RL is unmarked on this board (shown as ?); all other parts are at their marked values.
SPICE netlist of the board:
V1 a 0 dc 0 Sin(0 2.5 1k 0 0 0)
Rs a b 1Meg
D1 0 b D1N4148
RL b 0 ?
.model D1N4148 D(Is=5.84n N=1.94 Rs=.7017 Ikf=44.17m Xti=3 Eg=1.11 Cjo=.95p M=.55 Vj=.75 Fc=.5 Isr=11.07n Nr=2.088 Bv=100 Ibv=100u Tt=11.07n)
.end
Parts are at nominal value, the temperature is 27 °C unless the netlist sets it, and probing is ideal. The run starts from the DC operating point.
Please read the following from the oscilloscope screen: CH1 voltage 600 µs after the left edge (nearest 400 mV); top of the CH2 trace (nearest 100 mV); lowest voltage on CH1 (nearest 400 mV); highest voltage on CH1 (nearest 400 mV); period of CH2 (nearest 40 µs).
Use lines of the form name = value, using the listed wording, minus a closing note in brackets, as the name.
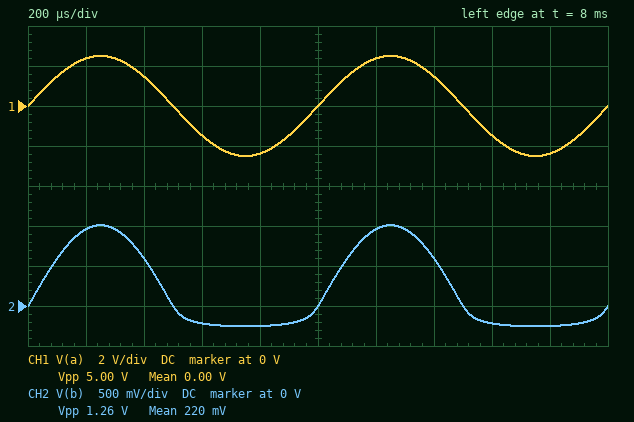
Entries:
CH1 voltage 600 µs after the left edge = -1.6 V
top of the CH2 trace = 1.0 V
lowest voltage on CH1 = -2.4 V
highest voltage on CH1 = 2.4 V
period of CH2 = 1.00 ms
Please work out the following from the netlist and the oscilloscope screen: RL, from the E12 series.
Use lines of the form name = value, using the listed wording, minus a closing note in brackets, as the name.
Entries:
RL, from the E12 series = 680 kΩ
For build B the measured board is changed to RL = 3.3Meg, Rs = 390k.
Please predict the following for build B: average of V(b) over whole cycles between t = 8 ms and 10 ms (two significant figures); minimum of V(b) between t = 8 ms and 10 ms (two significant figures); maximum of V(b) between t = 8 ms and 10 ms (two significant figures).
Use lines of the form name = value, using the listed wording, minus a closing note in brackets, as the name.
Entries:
average of V(b) over whole cycles between t = 8 ms and 10 ms = 580 mV
minimum of V(b) between t = 8 ms and 10 ms = -310 mV
maximum of V(b) between t = 8 ms and 10 ms = 2.2 V
